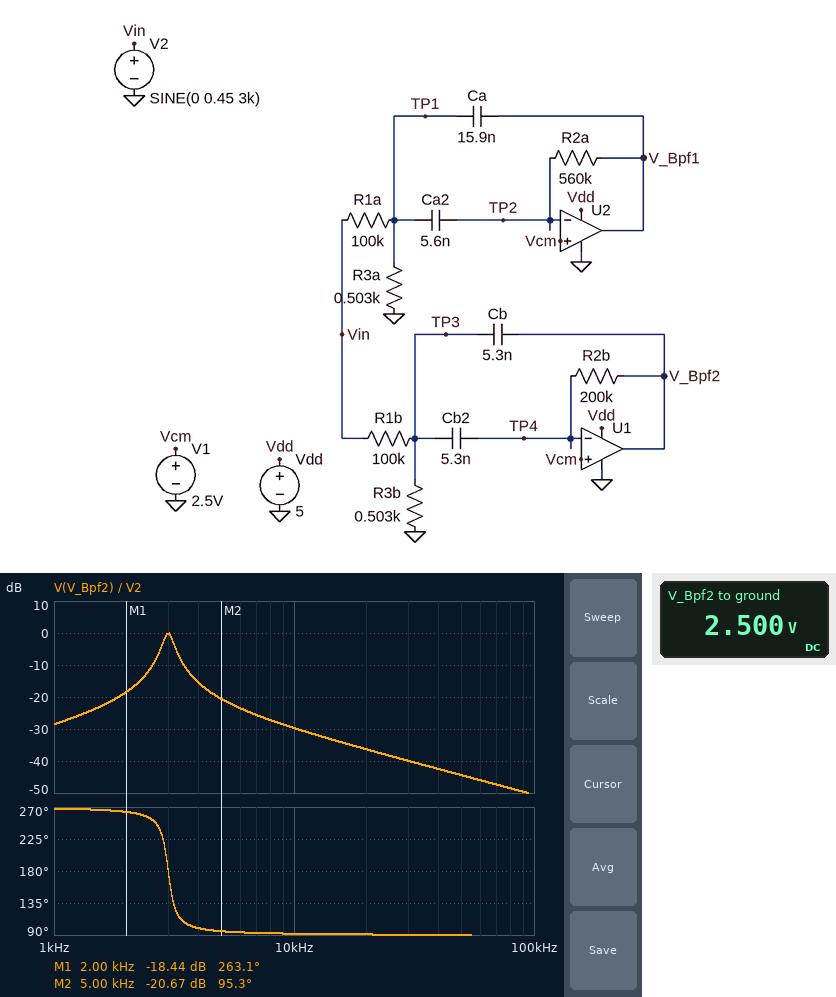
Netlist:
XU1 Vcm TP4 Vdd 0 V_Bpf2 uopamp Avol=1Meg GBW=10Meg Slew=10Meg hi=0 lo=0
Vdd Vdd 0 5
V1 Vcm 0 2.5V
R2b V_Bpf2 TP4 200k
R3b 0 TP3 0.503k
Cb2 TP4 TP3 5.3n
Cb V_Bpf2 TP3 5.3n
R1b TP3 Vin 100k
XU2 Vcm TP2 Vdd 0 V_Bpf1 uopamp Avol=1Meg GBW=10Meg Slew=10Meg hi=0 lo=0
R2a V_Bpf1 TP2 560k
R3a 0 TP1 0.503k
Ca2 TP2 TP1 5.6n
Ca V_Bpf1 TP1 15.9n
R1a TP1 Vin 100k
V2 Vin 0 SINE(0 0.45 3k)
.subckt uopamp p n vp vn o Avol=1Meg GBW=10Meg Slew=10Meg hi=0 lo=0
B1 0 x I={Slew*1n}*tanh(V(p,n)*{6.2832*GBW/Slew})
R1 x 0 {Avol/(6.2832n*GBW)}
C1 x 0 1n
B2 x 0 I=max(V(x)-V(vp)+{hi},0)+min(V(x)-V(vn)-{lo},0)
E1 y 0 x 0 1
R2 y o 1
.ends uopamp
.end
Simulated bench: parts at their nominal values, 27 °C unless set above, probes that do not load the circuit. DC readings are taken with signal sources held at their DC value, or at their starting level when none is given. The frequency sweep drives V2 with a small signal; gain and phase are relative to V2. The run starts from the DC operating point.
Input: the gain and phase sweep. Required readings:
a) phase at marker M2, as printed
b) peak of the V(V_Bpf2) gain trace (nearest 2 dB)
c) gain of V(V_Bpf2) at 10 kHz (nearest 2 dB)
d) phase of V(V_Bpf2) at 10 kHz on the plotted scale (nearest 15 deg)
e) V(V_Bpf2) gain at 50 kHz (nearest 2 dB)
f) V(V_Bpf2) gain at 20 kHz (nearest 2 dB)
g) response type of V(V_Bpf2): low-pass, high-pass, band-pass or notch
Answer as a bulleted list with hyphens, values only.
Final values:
- 95.3 deg
- 0 dB
- -30 dB
- 90 deg
- -44 dB
- -36 dB
- band-pass
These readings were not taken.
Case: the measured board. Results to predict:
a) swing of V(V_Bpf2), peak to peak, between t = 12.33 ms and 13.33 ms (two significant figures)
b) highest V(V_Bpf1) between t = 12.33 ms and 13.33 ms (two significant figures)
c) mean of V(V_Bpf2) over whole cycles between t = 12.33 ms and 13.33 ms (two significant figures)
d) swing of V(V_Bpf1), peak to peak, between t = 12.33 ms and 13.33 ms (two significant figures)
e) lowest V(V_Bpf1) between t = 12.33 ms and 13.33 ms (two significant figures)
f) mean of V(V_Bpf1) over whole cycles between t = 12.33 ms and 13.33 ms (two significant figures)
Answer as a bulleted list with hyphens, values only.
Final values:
- 900 mV
- 2.5 V
- 2.5 V
- 36 mV
- 2.5 V
- 2.5 V
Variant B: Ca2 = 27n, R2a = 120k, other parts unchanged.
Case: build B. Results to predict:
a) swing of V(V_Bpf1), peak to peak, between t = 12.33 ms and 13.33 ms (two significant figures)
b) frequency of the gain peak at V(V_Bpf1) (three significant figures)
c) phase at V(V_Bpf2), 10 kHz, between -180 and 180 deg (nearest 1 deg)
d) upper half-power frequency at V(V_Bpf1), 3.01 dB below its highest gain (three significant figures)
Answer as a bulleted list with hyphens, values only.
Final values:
- 34 mV
- 990 Hz
- 92 deg
- 1.06 kHz
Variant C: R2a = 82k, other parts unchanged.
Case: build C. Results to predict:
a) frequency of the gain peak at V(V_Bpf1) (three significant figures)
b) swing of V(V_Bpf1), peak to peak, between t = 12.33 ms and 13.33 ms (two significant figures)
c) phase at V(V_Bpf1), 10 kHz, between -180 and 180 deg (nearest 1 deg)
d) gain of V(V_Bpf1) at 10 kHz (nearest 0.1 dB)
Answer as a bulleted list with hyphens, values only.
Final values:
- 2.63 kHz
- 110 mV
- 93 deg
- -39.4 dB
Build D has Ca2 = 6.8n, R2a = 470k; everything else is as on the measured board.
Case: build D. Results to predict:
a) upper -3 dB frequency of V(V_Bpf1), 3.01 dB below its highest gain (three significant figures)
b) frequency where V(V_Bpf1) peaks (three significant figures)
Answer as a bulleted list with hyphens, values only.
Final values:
- 1.03 kHz
- 997 Hz
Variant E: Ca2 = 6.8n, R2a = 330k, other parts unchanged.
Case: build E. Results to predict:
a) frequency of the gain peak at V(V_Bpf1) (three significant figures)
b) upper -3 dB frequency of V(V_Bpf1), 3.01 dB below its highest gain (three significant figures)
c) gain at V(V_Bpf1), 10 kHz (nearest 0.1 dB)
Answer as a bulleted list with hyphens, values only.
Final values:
- 1.19 kHz
- 1.24 kHz
- -39.9 dB
